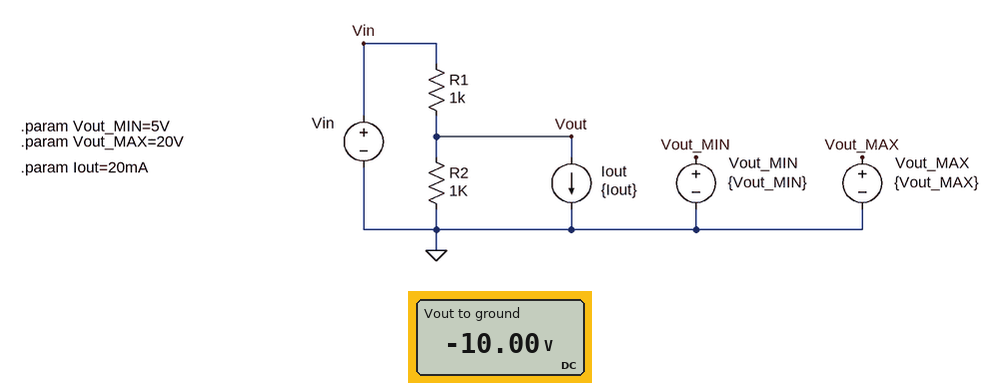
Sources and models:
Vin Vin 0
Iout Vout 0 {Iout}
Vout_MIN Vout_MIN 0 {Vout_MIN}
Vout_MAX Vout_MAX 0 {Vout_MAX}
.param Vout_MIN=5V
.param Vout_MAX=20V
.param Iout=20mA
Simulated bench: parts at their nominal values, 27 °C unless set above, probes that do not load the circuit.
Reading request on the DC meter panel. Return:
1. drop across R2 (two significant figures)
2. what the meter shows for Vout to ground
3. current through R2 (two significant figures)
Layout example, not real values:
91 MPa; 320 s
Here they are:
10 V; -10.00 V; 10 mA
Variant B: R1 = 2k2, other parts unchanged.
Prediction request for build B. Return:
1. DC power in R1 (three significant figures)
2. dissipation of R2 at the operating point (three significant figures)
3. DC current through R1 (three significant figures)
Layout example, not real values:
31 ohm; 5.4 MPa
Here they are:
85.9 mW; 189 mW; 6.25 mA
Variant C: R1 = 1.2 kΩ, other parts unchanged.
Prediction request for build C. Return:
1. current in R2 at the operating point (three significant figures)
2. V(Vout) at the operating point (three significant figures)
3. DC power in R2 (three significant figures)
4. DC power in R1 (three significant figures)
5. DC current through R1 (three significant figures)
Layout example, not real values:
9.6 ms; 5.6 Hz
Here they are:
10.9 mA; -10.9 V; 119 mW; 99.2 mW; 9.09 mA
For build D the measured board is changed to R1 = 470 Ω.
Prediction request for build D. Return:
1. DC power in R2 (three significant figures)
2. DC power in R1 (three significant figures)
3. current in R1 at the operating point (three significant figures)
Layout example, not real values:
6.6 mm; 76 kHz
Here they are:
40.9 mW; 87.0 mW; 13.6 mA
